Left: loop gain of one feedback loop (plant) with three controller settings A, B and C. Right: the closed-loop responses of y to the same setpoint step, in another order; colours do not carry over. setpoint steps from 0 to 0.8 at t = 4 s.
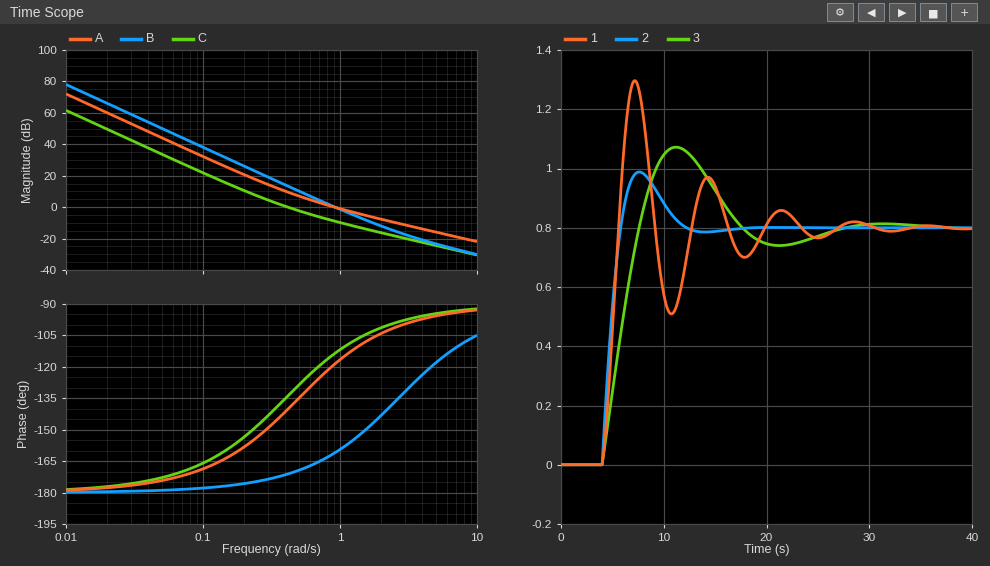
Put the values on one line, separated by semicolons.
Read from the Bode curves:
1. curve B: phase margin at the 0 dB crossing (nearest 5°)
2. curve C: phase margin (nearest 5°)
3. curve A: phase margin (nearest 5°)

20°; 45°; 60°
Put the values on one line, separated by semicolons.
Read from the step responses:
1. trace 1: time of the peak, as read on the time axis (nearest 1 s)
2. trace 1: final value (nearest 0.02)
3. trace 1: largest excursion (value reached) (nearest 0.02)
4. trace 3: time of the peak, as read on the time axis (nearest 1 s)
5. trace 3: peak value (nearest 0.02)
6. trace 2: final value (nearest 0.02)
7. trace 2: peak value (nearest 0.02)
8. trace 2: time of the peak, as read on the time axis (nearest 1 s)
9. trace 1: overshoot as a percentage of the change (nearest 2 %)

7 s; 0.80; 1.30; 11 s; 1.08; 0.80; 0.98; 8 s; 62 %
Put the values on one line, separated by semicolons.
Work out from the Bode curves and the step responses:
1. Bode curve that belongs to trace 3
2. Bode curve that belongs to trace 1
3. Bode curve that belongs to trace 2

C; B; A
